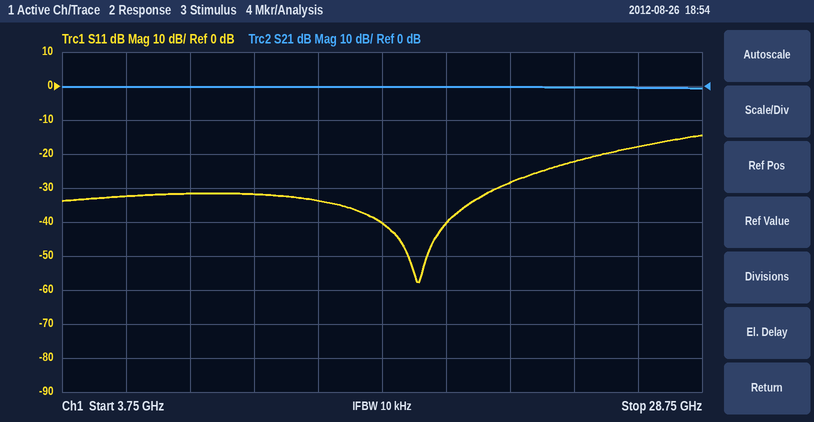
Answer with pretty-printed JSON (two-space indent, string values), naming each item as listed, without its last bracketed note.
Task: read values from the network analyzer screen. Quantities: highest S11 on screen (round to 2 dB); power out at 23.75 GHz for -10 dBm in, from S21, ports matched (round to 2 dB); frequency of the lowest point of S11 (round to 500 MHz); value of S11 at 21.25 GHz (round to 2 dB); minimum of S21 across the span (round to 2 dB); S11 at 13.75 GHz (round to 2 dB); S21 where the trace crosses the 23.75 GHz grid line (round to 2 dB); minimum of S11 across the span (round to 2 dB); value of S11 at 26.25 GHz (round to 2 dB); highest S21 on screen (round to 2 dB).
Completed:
{
  "highest S11 on screen": "-14 dB",
  "power out at 23.75 GHz for -10 dBm in, from S21, ports matched": "-10 dBm",
  "frequency of the lowest point of S11": "17.5 GHz",
  "value of S11 at 21.25 GHz": "-28 dB",
  "minimum of S21 across the span": "0 dB",
  "S11 at 13.75 GHz": "-34 dB",
  "S21 where the trace crosses the 23.75 GHz grid line": "0 dB",
  "minimum of S11 across the span": "-58 dB",
  "value of S11 at 26.25 GHz": "-18 dB",
  "highest S21 on screen": "0 dB"
}
